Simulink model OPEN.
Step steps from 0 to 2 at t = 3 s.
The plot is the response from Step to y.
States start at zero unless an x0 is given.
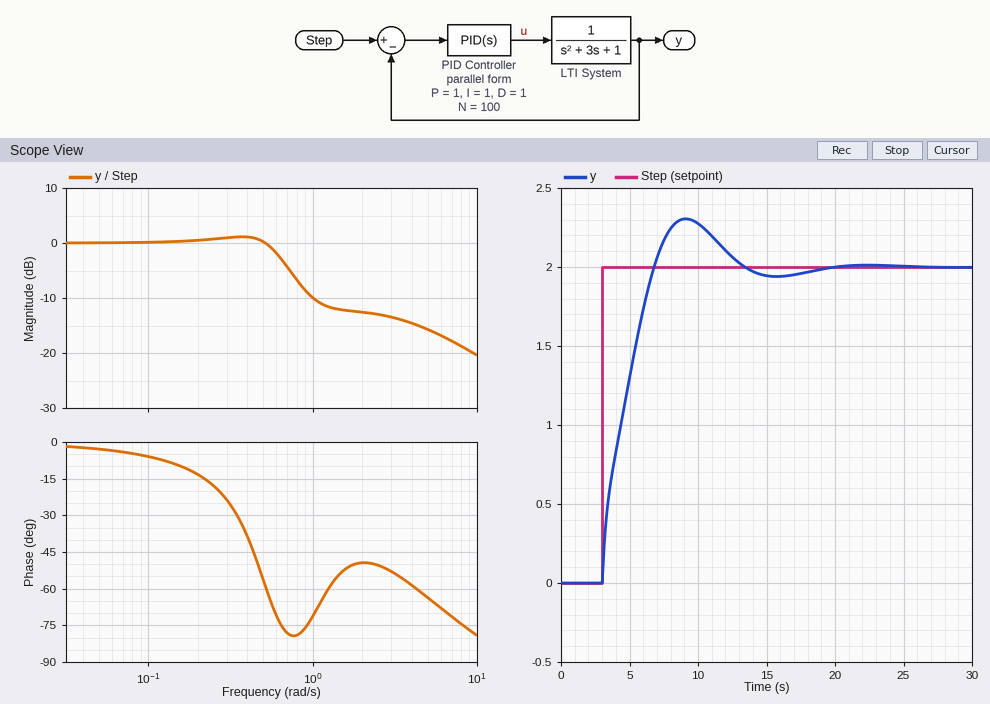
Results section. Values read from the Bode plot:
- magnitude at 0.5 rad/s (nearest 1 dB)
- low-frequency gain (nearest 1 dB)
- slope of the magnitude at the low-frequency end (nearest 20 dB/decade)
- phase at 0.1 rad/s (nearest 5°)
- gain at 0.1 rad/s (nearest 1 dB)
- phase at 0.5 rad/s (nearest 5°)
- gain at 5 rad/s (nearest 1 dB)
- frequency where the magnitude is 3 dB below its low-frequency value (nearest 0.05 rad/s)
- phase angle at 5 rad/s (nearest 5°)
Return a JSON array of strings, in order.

["0 dB", "0 dB", "0 dB/decade", "-5°", "0 dB", "-55°", "-16 dB", "0.65 rad/s", "-65°"]
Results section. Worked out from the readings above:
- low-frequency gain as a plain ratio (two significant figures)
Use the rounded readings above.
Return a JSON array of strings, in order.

["1.0"]
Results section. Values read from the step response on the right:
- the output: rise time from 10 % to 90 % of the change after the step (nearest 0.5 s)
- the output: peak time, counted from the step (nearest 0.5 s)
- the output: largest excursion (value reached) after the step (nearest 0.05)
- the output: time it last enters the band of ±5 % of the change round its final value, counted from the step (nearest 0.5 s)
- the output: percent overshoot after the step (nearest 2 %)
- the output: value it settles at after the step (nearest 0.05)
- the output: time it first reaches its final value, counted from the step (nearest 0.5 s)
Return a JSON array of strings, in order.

["3.0 s", "6.0 s", "2.30", "9.0 s", "16 %", "2.00", "4.0 s"]
